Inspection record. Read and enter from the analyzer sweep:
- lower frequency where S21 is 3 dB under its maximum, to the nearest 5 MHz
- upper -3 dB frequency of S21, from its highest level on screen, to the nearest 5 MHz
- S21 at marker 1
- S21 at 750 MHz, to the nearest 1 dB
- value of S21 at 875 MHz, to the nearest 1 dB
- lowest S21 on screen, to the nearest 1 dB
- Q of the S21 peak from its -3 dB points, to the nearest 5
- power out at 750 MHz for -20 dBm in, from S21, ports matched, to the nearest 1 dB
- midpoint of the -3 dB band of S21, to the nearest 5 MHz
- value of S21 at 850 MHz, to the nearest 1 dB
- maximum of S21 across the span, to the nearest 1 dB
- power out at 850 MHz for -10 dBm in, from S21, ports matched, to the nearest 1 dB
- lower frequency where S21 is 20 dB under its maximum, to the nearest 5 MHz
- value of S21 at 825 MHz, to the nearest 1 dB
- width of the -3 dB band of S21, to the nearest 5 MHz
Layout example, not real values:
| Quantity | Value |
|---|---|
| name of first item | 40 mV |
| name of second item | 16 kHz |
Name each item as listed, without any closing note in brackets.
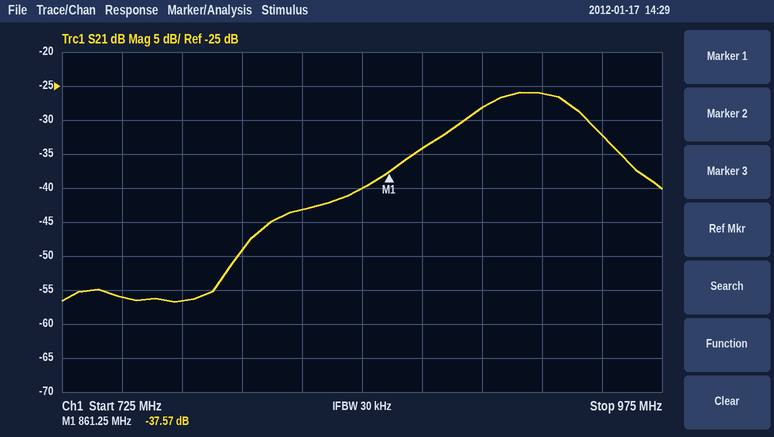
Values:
| Quantity | Value |
|---|---|
| lower frequency where S21 is 3 dB under its maximum, to the nearest 5 MHz | 895 MHz |
| upper -3 dB frequency of S21, from its highest level on screen, to the nearest 5 MHz | 940 MHz |
| S21 at marker 1 | -37.57 dB |
| S21 at 750 MHz, to the nearest 1 dB | -56 dB |
| value of S21 at 875 MHz, to the nearest 1 dB | -34 dB |
| lowest S21 on screen, to the nearest 1 dB | -57 dB |
| Q of the S21 peak from its -3 dB points, to the nearest 5 | 20 |
| power out at 750 MHz for -20 dBm in, from S21, ports matched, to the nearest 1 dB | -76 dBm |
| midpoint of the -3 dB band of S21, to the nearest 5 MHz | 920 MHz |
| value of S21 at 850 MHz, to the nearest 1 dB | -40 dB |
| maximum of S21 across the span, to the nearest 1 dB | -26 dB |
| power out at 850 MHz for -10 dBm in, from S21, ports matched, to the nearest 1 dB | -50 dBm |
| lower frequency where S21 is 20 dB under its maximum, to the nearest 5 MHz | 810 MHz |
| value of S21 at 825 MHz, to the nearest 1 dB | -43 dB |
| width of the -3 dB band of S21, to the nearest 5 MHz | 45 MHz |
